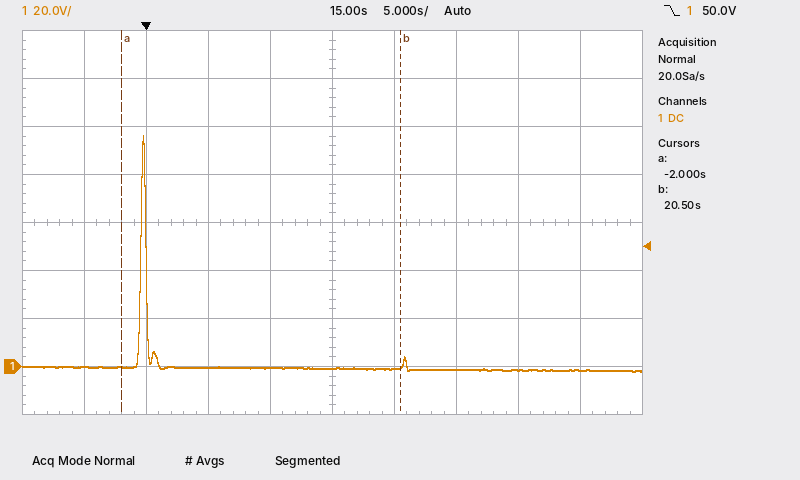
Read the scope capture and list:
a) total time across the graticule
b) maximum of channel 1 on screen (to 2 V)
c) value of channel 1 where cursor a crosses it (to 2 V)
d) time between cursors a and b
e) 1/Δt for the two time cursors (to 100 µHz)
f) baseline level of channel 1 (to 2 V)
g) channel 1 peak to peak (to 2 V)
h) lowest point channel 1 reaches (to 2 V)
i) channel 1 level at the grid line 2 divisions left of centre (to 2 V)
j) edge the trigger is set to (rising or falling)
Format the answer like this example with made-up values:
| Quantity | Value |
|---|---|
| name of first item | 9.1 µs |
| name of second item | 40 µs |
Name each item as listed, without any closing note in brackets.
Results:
| Quantity | Value |
|---|---|
| total time across the graticule | 50 s |
| maximum of channel 1 on screen | 96 V |
| value of channel 1 where cursor a crosses it | 0 V |
| time between cursors a and b | 22.5 s |
| 1/Δt for the two time cursors | 44.4 mHz |
| baseline level of channel 1 | 0 V |
| channel 1 peak to peak | 98 V |
| lowest point channel 1 reaches | -2 V |
| channel 1 level at the grid line 2 divisions left of centre | 0 V |
| edge the trigger is set to | falling |
